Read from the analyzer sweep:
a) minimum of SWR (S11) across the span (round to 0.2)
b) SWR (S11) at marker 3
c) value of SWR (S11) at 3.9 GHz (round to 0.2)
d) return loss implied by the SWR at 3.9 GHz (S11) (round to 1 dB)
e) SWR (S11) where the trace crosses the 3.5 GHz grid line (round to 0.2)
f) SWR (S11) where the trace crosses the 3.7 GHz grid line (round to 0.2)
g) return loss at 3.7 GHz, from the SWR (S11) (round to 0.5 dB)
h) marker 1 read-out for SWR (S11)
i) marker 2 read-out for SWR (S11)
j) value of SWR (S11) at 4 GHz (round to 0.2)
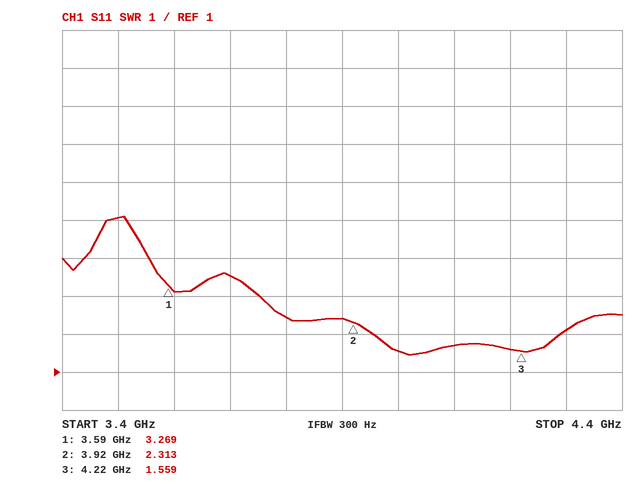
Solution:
1.4
1.559
2.4
8 dB
5.0
3.6
5.0 dB
3.269
2.313
1.6
